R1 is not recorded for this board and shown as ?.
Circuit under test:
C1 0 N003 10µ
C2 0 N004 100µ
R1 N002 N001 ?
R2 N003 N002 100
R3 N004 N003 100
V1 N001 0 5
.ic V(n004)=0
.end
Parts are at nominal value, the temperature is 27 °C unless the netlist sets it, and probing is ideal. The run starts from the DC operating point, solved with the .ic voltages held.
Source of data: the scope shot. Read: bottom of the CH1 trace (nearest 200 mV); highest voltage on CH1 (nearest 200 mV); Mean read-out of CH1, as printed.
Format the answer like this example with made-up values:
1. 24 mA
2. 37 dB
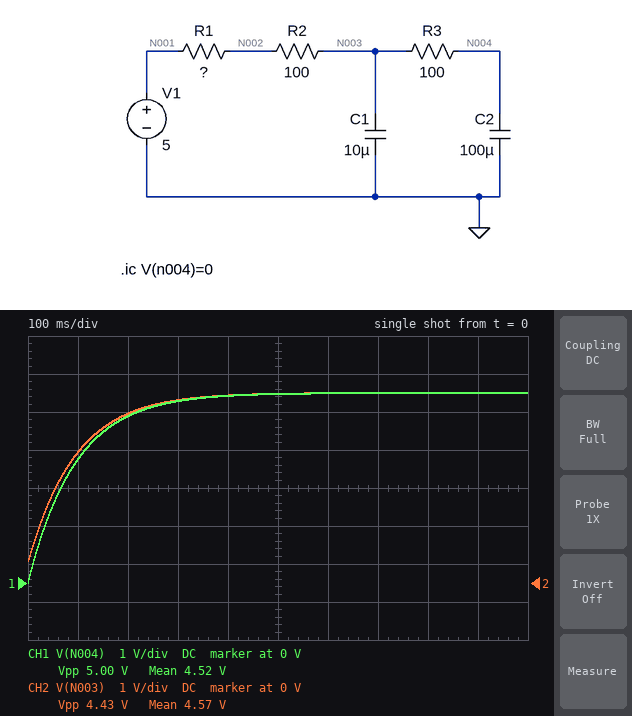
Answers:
1. 0 V
2. 5.0 V
3. 4.52 V
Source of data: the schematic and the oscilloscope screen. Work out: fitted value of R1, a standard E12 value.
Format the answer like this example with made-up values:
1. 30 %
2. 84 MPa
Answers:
1. 680 Ω
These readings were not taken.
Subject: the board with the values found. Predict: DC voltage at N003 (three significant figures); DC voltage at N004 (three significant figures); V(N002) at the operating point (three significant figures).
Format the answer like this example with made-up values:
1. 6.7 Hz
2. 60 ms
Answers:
1. 5.00 V
2. 5.00 V
3. 5.00 V
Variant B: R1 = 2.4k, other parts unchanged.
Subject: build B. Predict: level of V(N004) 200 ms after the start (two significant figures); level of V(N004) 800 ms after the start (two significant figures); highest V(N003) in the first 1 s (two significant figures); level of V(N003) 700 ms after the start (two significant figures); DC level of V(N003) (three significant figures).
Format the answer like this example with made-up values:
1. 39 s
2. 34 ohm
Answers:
1. 2.5 V
2. 4.7 V
3. 4.9 V
4. 4.6 V
5. 5.00 V
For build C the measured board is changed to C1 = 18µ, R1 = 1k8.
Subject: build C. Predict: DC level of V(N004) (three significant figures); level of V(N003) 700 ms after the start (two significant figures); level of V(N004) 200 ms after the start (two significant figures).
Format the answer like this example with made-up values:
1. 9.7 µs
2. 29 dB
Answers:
1. 5.00 V
2. 4.8 V
3. 2.9 V
